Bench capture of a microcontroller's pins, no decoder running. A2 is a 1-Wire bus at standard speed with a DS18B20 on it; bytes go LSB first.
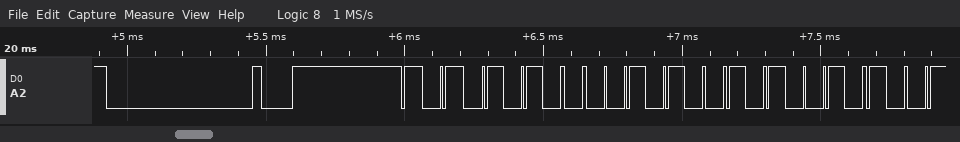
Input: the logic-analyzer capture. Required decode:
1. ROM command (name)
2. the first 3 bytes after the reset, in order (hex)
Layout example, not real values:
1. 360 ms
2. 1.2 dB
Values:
1. Match ROM
2. 55 28 A5
